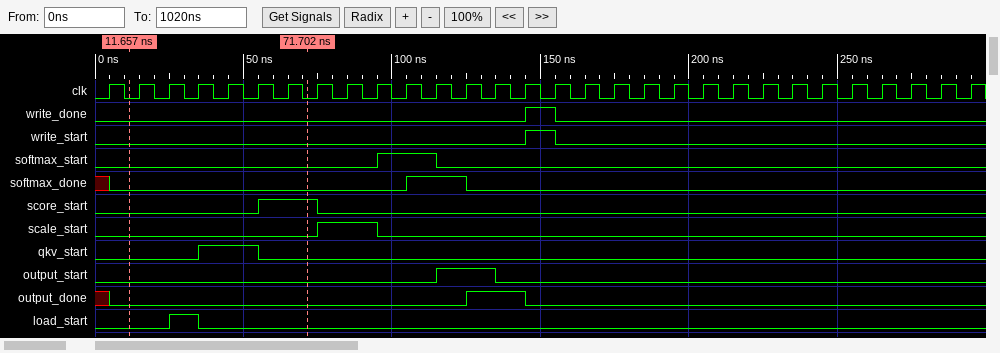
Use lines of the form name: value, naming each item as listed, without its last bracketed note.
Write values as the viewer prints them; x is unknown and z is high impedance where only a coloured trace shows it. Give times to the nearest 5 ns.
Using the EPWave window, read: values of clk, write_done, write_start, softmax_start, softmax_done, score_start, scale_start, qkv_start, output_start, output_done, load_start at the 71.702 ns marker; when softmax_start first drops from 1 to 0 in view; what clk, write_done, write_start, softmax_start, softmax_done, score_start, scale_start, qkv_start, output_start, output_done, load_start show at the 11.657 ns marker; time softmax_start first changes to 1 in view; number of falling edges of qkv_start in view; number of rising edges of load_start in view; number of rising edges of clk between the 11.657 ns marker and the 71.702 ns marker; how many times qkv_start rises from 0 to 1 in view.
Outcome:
values of clk, write_done, write_start, softmax_start, softmax_done, score_start, scale_start, qkv_start, output_start, output_done, load_start at the 71.702 ns marker: clk=0, write_done=0, write_start=0, softmax_start=0, softmax_done=0, score_start=1, scale_start=0, qkv_start=0, output_start=0, output_done=0, load_start=0
when softmax_start first drops from 1 to 0 in view: 115 ns
what clk, write_done, write_start, softmax_start, softmax_done, score_start, scale_start, qkv_start, output_start, output_done, load_start show at the 11.657 ns marker: clk=0, write_done=0, write_start=0, softmax_start=0, softmax_done=0, score_start=0, scale_start=0, qkv_start=0, output_start=0, output_done=0, load_start=0
time softmax_start first changes to 1 in view: 95 ns
number of falling edges of qkv_start in view: 1
number of rising edges of load_start in view: 1
number of rising edges of clk between the 11.657 ns marker and the 71.702 ns marker: 6
how many times qkv_start rises from 0 to 1 in view: 1
